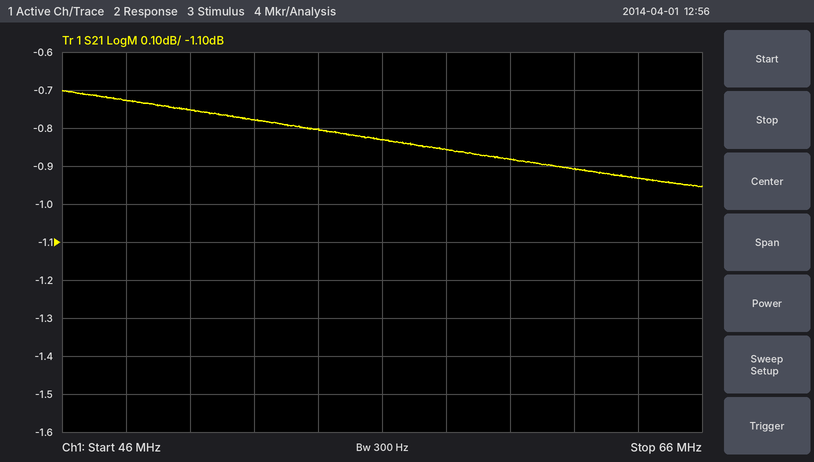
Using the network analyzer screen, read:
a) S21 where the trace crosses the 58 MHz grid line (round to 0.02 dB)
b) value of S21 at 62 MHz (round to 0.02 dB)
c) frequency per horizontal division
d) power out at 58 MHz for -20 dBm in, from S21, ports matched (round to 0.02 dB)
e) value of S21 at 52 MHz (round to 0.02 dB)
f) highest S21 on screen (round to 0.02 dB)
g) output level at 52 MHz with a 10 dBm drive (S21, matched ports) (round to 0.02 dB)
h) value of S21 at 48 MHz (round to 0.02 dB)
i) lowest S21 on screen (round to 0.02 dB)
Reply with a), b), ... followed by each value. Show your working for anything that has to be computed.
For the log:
a) -0.86 dB
b) -0.90 dB
c) 2 MHz
d) -20 dBm + (-0.86 dB) = -20.86 dBm
e) -0.78 dB
f) -0.70 dB
g) 10 dBm + (-0.78 dB) = 9.22 dBm
h) -0.72 dB
i) -0.96 dB
